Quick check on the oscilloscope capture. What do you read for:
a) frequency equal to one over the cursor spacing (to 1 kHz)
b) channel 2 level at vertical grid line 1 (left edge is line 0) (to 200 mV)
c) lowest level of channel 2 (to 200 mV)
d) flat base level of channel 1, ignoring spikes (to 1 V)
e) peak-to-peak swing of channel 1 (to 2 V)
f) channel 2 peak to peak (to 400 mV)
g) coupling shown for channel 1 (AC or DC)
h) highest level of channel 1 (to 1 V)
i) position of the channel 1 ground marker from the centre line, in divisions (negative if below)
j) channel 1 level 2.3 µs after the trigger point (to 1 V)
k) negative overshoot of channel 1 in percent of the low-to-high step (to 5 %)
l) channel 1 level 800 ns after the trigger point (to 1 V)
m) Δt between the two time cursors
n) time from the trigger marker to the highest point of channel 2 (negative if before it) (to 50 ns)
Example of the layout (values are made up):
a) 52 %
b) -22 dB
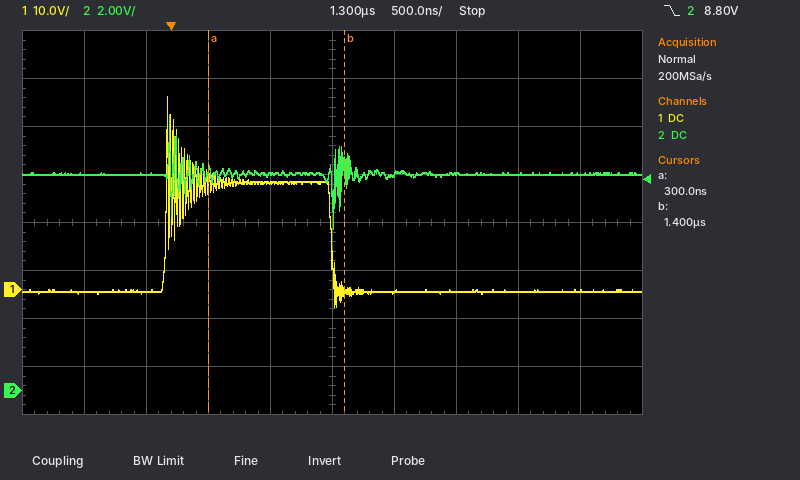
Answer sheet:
a) 909 kHz
b) 9.0 V
c) 6.8 V
d) 0 V
e) 44 V
f) 4.8 V
g) DC
h) 40 V
i) -1.4 div
j) 0 V
k) 15 %
l) 22 V
m) 1.10 µs
n) 0 ns
